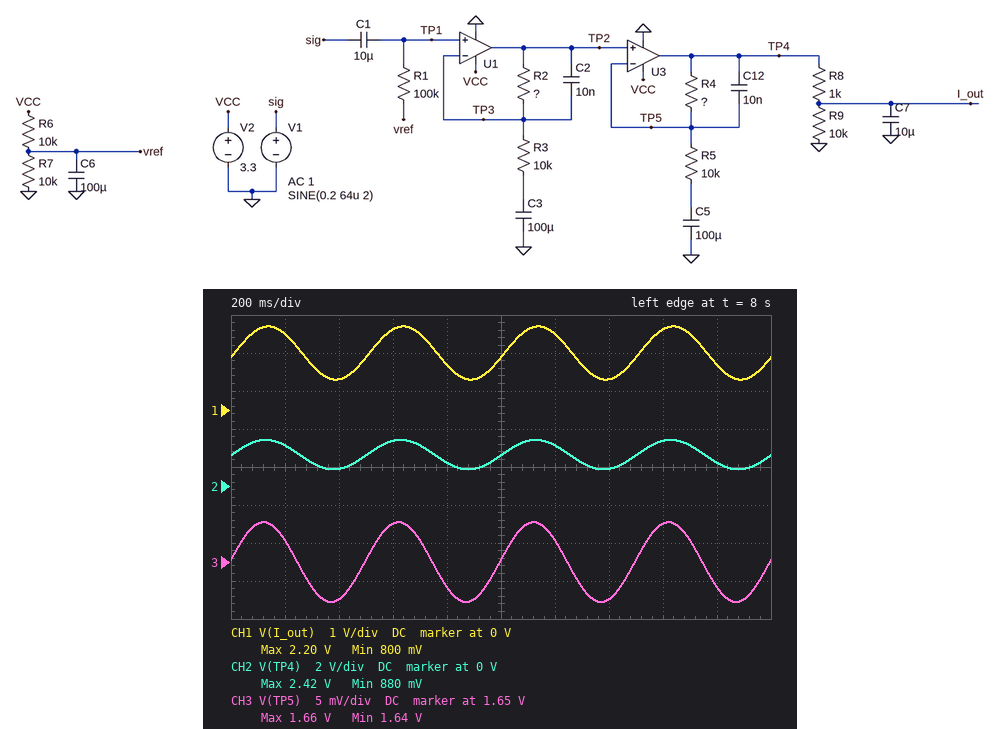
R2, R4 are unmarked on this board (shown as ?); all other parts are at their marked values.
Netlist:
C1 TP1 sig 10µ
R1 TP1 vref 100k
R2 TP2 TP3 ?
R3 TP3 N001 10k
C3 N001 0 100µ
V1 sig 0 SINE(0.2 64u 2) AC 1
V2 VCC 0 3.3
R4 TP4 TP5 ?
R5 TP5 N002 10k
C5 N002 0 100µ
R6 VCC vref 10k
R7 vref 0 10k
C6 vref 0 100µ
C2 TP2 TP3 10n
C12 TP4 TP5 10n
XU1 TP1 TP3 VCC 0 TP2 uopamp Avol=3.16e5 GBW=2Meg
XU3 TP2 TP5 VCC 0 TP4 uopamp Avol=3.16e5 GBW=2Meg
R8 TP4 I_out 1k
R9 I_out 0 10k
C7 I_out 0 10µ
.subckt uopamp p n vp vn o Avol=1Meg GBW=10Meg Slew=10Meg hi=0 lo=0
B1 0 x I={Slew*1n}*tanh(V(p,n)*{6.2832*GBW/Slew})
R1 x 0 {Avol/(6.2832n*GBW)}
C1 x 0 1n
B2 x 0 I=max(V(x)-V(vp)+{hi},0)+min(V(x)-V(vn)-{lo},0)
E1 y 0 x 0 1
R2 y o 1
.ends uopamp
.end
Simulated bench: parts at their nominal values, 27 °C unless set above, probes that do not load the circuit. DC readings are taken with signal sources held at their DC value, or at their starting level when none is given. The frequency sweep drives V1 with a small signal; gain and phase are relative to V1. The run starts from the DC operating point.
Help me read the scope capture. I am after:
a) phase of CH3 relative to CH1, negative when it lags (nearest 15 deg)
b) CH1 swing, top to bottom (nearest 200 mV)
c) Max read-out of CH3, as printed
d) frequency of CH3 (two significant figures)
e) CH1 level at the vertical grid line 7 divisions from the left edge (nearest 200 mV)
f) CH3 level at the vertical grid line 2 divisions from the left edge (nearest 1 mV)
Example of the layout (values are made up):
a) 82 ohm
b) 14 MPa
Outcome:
a) 15 deg
b) 1.4 V
c) 1.66 V
d) 2.0 Hz
e) 800 mV
f) 1.645 V
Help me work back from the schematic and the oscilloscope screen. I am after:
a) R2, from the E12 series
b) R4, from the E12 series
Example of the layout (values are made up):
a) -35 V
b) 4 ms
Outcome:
a) 820 kΩ
b) 1.5 MΩ
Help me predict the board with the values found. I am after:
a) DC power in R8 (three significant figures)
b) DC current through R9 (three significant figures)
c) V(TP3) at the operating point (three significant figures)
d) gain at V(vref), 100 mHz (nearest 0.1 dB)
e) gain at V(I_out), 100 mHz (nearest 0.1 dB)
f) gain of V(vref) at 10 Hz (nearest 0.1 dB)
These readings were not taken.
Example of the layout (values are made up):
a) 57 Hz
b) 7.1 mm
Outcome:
a) 22.5 µW
b) 150 µA
c) 1.65 V
d) -32.1 dB
e) 64.9 dB
f) -56.0 dB
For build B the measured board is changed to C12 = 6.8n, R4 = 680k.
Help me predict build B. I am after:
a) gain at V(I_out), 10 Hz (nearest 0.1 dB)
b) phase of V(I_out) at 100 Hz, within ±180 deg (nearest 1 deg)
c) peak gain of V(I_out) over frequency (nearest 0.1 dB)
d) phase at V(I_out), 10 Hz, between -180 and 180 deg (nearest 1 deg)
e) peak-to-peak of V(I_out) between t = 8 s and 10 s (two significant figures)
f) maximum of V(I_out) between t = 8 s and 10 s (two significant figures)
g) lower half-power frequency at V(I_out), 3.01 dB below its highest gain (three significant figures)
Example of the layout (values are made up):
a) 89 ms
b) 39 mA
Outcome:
a) 71.7 dB
b) 136 deg
c) 74.1 dB
d) -70 deg
e) 650 mV
f) 1.8 V
g) 303 mHz
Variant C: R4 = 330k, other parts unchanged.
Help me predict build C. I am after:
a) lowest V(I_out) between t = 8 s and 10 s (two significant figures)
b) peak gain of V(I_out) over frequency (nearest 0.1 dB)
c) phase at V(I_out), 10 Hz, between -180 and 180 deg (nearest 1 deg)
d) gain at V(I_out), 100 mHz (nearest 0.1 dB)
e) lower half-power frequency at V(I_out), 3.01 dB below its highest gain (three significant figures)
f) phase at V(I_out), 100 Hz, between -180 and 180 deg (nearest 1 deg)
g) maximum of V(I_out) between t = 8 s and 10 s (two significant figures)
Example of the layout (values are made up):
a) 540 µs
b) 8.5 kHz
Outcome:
a) 1.3 V
b) 68.0 dB
c) -65 deg
d) 52.0 dB
e) 303 mHz
f) 144 deg
g) 1.7 V
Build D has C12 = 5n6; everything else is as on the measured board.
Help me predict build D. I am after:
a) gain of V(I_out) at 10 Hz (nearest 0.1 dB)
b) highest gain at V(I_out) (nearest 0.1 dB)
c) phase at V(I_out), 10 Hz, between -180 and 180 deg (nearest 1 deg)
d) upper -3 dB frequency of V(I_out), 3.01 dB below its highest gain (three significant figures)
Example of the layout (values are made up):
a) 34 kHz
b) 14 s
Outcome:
a) 77.8 dB
b) 80.9 dB
c) -82 deg
d) 9.86 Hz
